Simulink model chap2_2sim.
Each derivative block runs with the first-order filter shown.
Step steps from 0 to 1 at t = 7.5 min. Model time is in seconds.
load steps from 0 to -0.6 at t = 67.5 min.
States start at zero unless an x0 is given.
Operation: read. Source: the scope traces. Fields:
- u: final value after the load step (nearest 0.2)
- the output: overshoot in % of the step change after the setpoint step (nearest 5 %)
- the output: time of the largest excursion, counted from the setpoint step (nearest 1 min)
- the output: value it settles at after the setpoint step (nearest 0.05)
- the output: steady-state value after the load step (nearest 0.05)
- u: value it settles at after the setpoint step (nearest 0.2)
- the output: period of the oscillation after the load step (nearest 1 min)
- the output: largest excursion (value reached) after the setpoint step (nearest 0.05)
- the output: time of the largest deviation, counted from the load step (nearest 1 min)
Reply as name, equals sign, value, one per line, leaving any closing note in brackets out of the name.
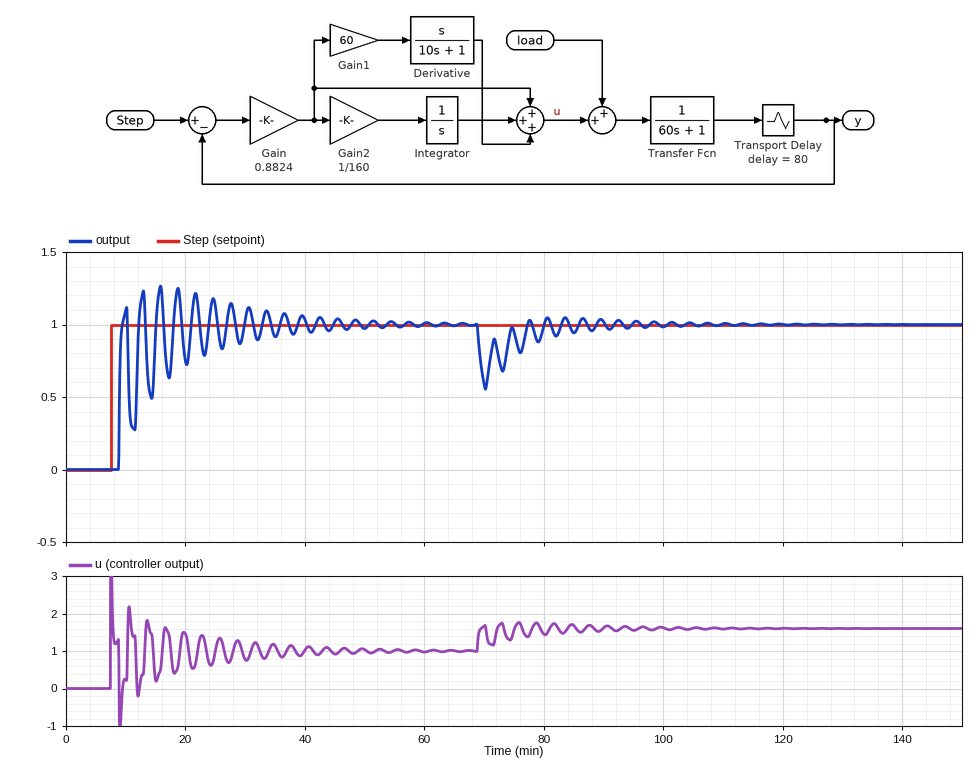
u: final value after the load step = 1.6
the output: overshoot in % of the step change after the setpoint step = 25 %
the output: time of the largest excursion, counted from the setpoint step = 8 min
the output: value it settles at after the setpoint step = 1.00
the output: steady-state value after the load step = 1.00
u: value it settles at after the setpoint step = 1.0
the output: period of the oscillation after the load step = 3 min
the output: largest excursion (value reached) after the setpoint step = 1.25
the output: time of the largest deviation, counted from the load step = 3 min
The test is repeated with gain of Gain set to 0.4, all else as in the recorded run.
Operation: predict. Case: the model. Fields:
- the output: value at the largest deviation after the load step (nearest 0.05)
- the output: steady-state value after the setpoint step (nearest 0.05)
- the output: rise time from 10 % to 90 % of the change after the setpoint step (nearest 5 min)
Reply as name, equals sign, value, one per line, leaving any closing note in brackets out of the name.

the output: value at the largest deviation after the load step = 0.55
the output: steady-state value after the setpoint step = 1.00
the output: rise time from 10 % to 90 % of the change after the setpoint step = 15 min
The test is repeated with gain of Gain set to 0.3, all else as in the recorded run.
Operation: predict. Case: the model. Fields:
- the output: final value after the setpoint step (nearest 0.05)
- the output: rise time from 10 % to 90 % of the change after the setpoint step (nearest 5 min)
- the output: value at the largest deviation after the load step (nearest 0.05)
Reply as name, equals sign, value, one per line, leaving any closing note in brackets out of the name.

the output: final value after the setpoint step = 1.00
the output: rise time from 10 % to 90 % of the change after the setpoint step = 20 min
the output: value at the largest deviation after the load step = 0.55
